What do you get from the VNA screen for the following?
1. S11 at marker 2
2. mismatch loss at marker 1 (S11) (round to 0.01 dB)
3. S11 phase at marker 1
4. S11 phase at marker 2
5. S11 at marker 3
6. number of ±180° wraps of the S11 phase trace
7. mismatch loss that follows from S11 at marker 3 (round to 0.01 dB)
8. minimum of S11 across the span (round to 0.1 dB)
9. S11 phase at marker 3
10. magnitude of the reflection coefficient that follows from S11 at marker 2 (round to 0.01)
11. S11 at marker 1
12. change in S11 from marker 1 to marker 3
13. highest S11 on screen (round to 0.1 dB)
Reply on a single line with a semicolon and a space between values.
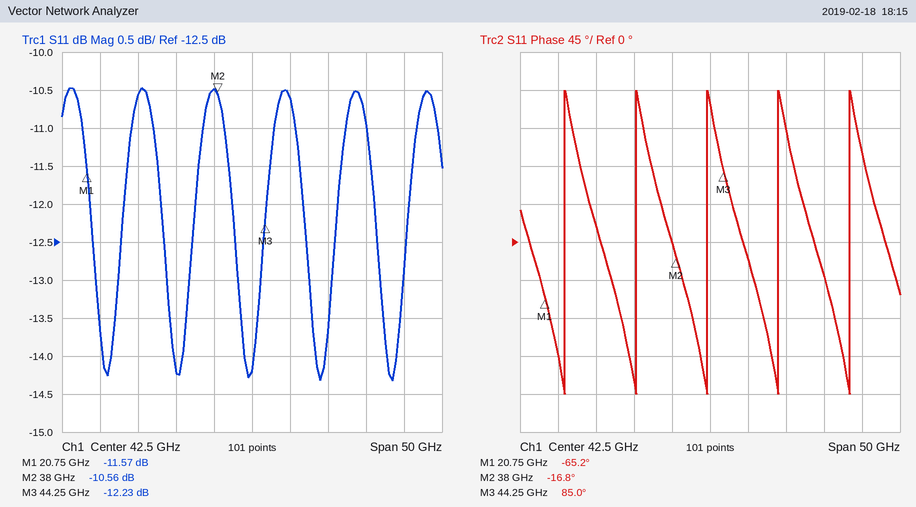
-10.56 dB; 0.31 dB; -65.2°; -16.8°; -12.23 dB; 5; 0.27 dB; -14.3 dB; 85.0°; 0.30; -11.57 dB; -0.66 dB; -10.5 dB
